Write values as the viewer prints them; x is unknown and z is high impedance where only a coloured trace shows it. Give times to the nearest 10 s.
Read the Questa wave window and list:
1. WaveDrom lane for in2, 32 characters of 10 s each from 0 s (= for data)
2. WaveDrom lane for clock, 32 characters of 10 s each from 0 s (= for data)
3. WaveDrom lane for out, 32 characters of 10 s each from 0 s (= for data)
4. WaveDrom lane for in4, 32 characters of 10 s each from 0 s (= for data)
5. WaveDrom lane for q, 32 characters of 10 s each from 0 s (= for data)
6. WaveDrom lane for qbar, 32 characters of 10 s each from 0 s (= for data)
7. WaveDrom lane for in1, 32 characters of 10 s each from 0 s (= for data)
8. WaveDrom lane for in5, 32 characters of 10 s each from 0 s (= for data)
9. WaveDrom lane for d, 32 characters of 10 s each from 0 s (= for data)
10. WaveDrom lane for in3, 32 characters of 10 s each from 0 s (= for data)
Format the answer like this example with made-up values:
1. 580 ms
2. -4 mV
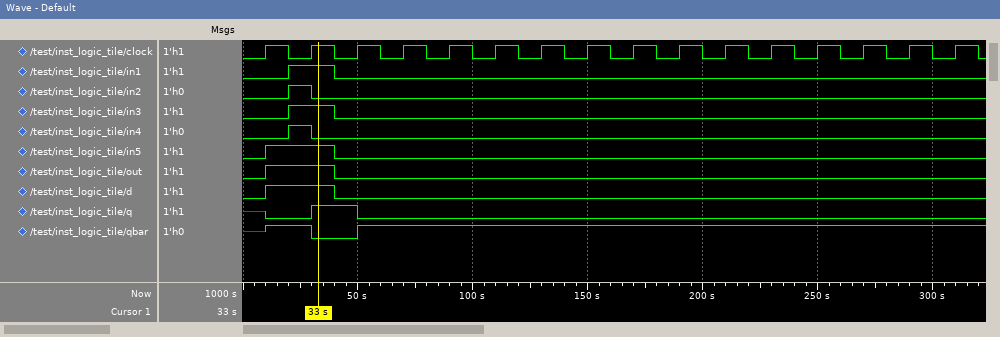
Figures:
1. {name: 'in2', wave: '0.10............................'}
2. {name: 'clock', wave: '01010101010101010101010101010101'}
3. {name: 'out', wave: '01..0...........................'}
4. {name: 'in4', wave: '0.10............................'}
5. {name: 'q', wave: 'x0.1.0..........................'}
6. {name: 'qbar', wave: 'x1.0.1..........................'}
7. {name: 'in1', wave: '0.1.0...........................'}
8. {name: 'in5', wave: '01..0...........................'}
9. {name: 'd', wave: '01..0...........................'}
10. {name: 'in3', wave: '0.1.0...........................'}
